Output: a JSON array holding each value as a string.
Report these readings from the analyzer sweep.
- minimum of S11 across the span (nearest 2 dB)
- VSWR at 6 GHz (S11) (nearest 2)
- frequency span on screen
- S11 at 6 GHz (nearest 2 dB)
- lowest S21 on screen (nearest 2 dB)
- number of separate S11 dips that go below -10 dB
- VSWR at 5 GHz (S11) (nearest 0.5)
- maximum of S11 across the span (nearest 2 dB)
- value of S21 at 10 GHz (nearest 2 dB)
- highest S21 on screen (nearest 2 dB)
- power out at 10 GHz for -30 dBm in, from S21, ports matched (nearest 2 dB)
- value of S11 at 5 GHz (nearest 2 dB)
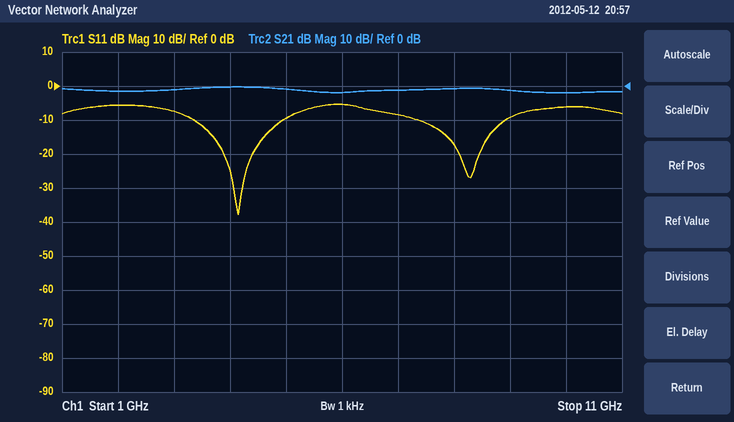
["-38 dB", "4", "10 GHz", "-6 dB", "-2 dB", "2", "2.0", "-6 dB", "-2 dB", "0 dB", "-32 dBm", "-10 dB"]
